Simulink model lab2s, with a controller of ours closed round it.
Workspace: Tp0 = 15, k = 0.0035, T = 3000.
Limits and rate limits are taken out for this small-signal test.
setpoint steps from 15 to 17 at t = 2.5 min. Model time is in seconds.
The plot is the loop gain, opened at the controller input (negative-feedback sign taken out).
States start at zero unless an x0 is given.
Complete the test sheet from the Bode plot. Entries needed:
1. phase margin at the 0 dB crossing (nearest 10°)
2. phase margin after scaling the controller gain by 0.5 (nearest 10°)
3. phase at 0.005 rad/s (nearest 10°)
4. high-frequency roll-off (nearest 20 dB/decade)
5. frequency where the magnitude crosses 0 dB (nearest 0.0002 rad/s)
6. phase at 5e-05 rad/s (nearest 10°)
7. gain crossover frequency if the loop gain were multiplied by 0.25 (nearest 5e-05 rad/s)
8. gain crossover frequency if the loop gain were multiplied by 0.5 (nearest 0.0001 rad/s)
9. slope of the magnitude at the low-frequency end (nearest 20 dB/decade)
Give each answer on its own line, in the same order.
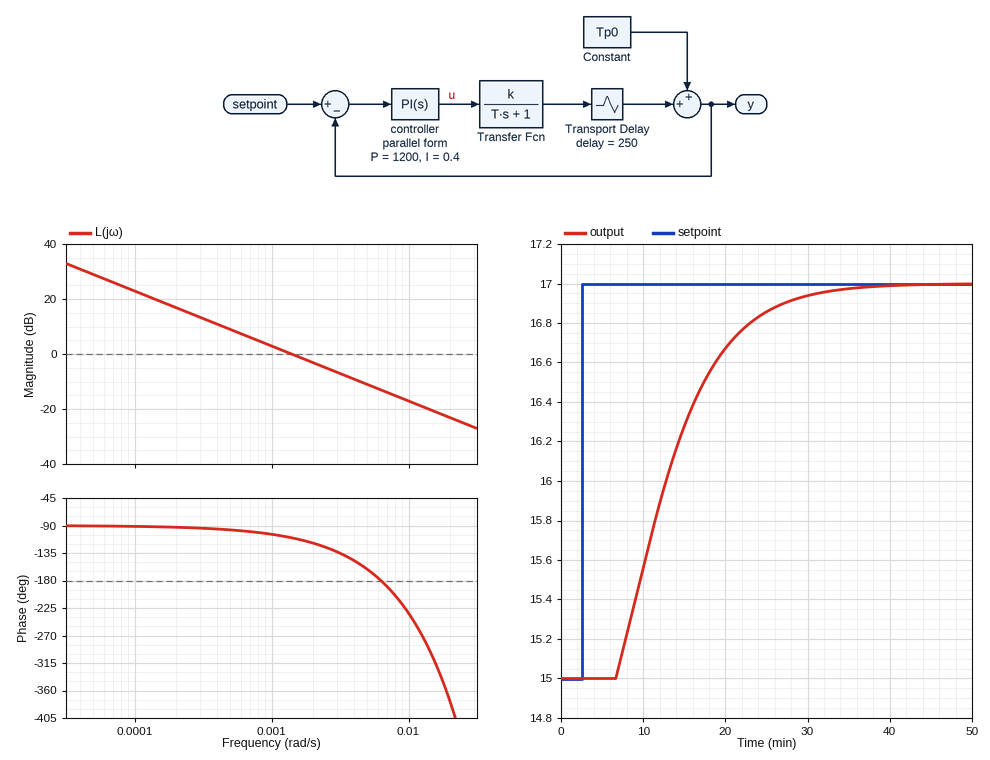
70°
80°
-160°
-20 dB/decade
0.0014 rad/s
-90°
0.00035 rad/s
0.0007 rad/s
-20 dB/decade
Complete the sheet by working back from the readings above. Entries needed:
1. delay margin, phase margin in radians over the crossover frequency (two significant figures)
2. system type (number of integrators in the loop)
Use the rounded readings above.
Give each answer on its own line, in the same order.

870 s
1
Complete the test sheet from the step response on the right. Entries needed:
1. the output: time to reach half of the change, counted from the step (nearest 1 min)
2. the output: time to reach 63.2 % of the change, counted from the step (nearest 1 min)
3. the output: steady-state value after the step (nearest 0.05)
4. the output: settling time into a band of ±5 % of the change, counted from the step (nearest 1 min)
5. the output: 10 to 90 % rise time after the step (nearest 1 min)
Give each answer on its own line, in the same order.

10 min
12 min
17.00
25 min
15 min
